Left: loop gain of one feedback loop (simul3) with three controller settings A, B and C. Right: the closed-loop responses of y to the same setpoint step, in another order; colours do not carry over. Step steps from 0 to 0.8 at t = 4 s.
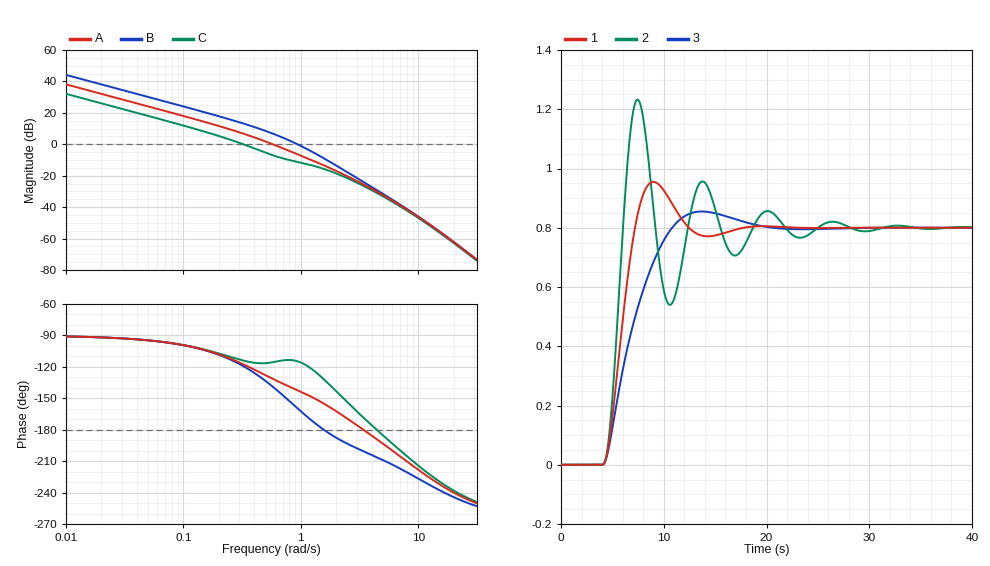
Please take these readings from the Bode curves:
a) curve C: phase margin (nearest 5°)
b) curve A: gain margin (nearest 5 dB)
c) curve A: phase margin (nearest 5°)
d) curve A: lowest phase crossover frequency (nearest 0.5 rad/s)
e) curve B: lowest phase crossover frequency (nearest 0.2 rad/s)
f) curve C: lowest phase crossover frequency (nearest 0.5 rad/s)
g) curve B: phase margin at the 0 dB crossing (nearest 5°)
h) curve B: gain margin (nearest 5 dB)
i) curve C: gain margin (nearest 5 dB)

65°
25 dB
50°
3.5 rad/s
1.6 rad/s
4.5 rad/s
20°
10 dB
30 dB
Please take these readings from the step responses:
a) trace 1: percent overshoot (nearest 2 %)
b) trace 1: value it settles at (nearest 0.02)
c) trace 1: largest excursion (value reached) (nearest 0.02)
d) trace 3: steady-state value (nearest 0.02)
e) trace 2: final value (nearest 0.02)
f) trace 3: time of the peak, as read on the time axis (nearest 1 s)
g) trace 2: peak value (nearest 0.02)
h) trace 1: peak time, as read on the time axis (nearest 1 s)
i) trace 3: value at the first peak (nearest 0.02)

20 %
0.80
0.96
0.80
0.80
14 s
1.24
9 s
0.86
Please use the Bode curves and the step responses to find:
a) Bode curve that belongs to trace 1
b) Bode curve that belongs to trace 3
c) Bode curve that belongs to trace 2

A
C
B
